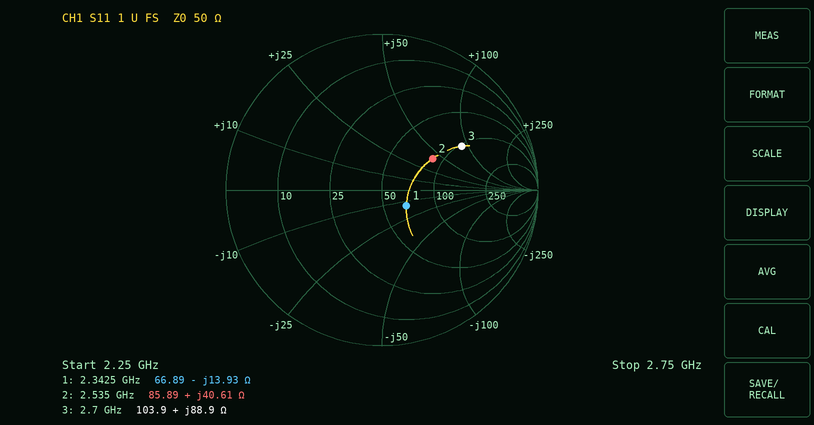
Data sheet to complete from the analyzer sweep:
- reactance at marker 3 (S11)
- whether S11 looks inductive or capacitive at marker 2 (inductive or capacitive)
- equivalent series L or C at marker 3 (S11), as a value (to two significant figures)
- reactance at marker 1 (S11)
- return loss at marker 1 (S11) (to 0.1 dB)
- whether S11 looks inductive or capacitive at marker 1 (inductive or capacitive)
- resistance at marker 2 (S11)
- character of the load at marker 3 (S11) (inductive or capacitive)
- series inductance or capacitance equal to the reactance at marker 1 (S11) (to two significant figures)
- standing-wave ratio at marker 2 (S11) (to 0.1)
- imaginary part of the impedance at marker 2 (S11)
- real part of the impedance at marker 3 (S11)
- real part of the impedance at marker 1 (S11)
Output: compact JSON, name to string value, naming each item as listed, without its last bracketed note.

{"reactance at marker 3": "+88.9 Ω", "whether S11 looks inductive or capacitive at marker 2": "inductive", "equivalent series L or C at marker 3 (S11), as a value": "5.2 nH", "reactance at marker 1": "-13.93 Ω", "return loss at marker 1 (S11)": "14.6 dB", "whether S11 looks inductive or capacitive at marker 1": "capacitive", "resistance at marker 2": "85.89 Ω", "character of the load at marker 3 (S11)": "inductive", "series inductance or capacitance equal to the reactance at marker 1 (S11)": "4.9 pF", "standing-wave ratio at marker 2 (S11)": "2.2", "imaginary part of the impedance at marker 2": "+40.61 Ω", "real part of the impedance at marker 3": "103.9 Ω", "real part of the impedance at marker 1": "66.89 Ω"}
